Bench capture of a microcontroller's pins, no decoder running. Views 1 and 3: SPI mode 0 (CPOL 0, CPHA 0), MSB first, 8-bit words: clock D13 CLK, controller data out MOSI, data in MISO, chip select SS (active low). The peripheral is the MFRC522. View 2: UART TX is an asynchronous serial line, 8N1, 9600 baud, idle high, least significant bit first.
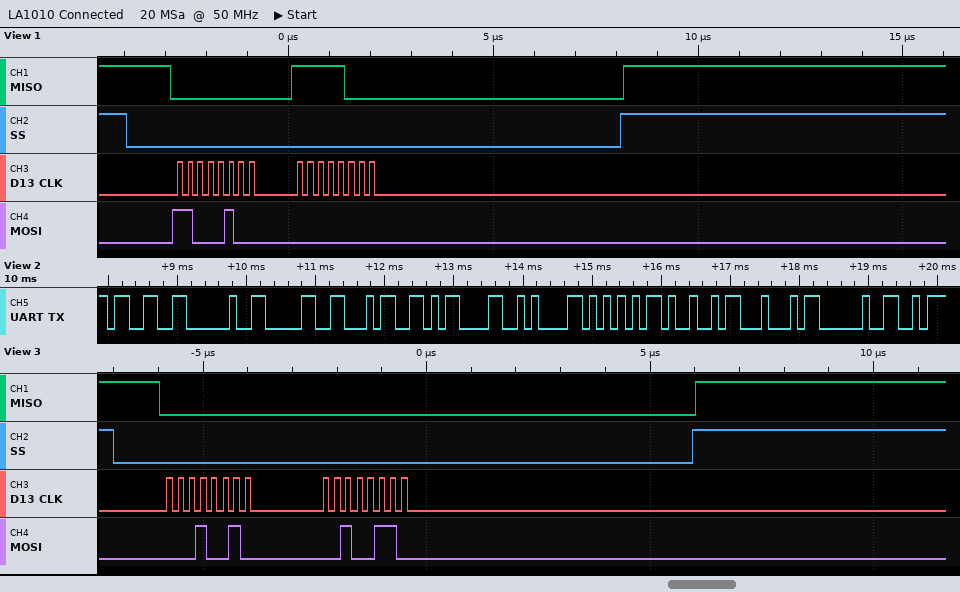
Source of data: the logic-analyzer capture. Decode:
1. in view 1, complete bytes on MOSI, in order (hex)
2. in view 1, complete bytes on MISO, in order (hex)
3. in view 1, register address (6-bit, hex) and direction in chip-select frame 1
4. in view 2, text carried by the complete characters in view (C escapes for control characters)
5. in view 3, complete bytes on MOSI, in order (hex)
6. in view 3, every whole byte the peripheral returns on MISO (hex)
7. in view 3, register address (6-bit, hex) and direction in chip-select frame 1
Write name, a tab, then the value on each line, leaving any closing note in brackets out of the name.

in view 1, complete bytes on MOSI, in order	0xC4 0x00
in view 1, complete bytes on MISO, in order	0x00 0xF8
in view 1, register address (6-bit, hex) and direction in chip-select frame 1	0x22 read
in view 2, text carried by the complete characters in view	"3 04\r\nUID "
in view 3, complete bytes on MOSI, in order	12 26
in view 3, every whole byte the peripheral returns on MISO	00 00
in view 3, register address (6-bit, hex) and direction in chip-select frame 1	0x09 write
